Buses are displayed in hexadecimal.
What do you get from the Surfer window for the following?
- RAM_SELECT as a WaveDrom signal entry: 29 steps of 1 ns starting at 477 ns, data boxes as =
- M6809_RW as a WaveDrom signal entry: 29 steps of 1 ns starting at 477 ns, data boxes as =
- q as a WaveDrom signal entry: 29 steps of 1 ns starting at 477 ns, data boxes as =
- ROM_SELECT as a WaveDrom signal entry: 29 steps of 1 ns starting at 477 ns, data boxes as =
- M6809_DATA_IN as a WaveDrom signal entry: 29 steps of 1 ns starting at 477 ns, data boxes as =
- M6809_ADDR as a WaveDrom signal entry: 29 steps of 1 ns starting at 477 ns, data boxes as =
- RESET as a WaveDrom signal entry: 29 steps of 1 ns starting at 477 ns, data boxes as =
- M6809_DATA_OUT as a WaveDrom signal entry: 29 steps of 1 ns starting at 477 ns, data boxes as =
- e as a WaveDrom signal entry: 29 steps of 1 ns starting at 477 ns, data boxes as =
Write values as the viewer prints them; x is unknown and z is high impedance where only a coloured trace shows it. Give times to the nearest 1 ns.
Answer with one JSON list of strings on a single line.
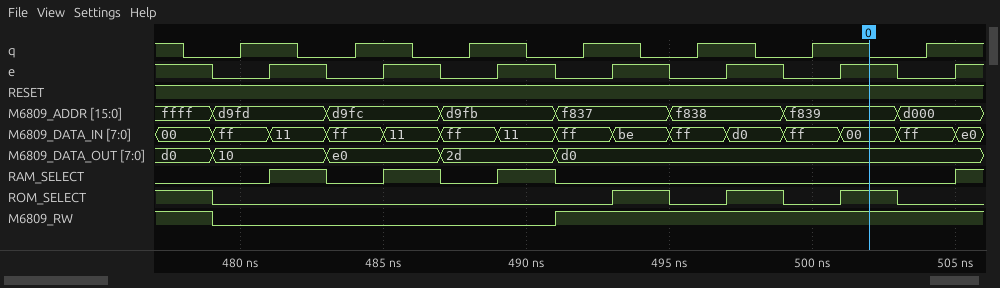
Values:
["{name: 'RAM_SELECT', wave: '0...1.0.1.0.1.0.............1'}", "{name: 'M6809_RW', wave: '1.0...........1..............'}", "{name: 'q', wave: '10.1.0.1.0.1.0.1.0.1.0.1.0.1.'}", "{name: 'ROM_SELECT', wave: '1.0.............1.0.1.0.1.0..'}", "{name: 'M6809_DATA_IN', wave: '=.=.=.=.=.=.=.=.=.=.=.=.=.=.=', data: '00 ff 11 ff 11 ff 11 ff be ff d0 ff 00 ff e0'}", "{name: 'M6809_ADDR', wave: '=.=...=...=...=...=...=...=..', data: 'ffff d9fd d9fc d9fb f837 f838 f839 d000'}", "{name: 'RESET', wave: '1............................'}", "{name: 'M6809_DATA_OUT', wave: '=.=...=...=...=..............', data: 'd0 10 e0 2d d0'}", "{name: 'e', wave: '1.0.1.0.1.0.1.0.1.0.1.0.1.0.1'}"]
